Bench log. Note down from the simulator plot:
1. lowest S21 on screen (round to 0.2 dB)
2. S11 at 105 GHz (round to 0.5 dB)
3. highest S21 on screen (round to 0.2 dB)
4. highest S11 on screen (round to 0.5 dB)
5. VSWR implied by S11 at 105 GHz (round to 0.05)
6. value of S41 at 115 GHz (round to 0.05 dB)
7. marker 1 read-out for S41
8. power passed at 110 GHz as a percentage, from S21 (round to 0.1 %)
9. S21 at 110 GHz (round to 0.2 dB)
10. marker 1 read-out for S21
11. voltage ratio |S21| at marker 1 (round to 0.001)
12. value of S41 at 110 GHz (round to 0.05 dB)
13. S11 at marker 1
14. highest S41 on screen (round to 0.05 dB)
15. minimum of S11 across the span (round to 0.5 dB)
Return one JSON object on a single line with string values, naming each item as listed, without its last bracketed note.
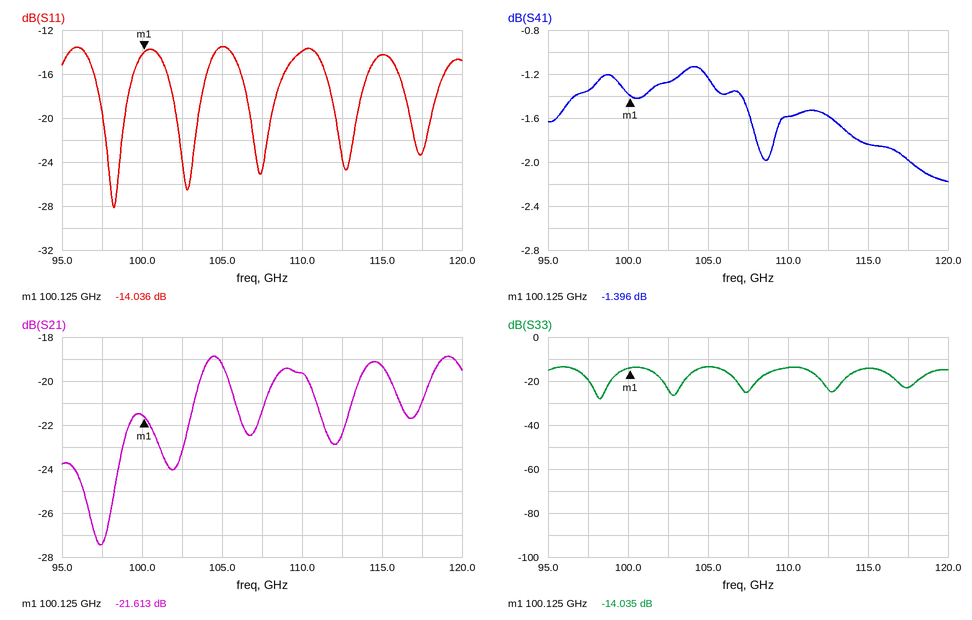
{"lowest S21 on screen": "-27.4 dB", "S11 at 105 GHz": "-13.5 dB", "highest S21 on screen": "-18.8 dB", "highest S11 on screen": "-13.5 dB", "VSWR implied by S11 at 105 GHz": "1.55", "value of S41 at 115 GHz": "-1.85 dB", "marker 1 read-out for S41": "-1.396 dB", "power passed at 110 GHz as a percentage, from S21": "1.1 %", "S21 at 110 GHz": "-19.6 dB", "marker 1 read-out for S21": "-21.613 dB", "voltage ratio |S21| at marker 1": "0.083", "value of S41 at 110 GHz": "-1.60 dB", "S11 at marker 1": "-14.036 dB", "highest S41 on screen": "-1.15 dB", "minimum of S11 across the span": "-28.0 dB"}
